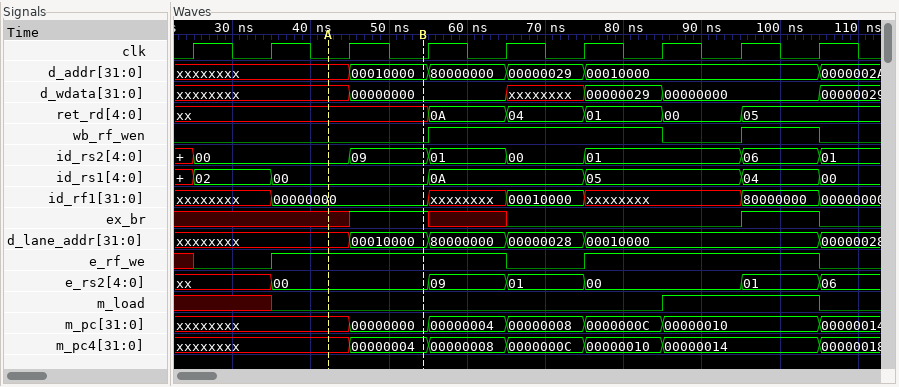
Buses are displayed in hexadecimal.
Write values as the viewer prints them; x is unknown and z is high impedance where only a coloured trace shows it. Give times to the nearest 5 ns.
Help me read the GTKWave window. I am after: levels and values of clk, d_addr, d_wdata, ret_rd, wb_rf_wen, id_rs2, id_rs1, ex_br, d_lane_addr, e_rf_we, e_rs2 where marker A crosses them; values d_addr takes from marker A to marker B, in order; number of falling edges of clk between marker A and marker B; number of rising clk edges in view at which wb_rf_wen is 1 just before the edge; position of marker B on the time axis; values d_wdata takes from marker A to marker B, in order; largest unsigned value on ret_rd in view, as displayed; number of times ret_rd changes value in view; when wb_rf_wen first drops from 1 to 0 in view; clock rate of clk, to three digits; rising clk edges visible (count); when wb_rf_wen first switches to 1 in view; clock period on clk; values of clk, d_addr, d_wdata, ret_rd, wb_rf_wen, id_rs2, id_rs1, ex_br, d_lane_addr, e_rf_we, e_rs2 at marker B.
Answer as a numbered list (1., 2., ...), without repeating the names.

1. clk=0, d_addr=xxxxxxxx, d_wdata=xxxxxxxx, ret_rd=xx, wb_rf_wen=0, id_rs2=00, id_rs1=00, ex_br=x, d_lane_addr=xxxxxxxx, e_rf_we=1, e_rs2=00
2. xxxxxxxx, 00010000
3. 1
4. 4
5. 55 ns
6. xxxxxxxx, 00000000
7. 0A
8. 5
9. 85 ns
10. 100 MHz
11. 9
12. 55 ns
13. 10 ns
14. clk=0, d_addr=00010000, d_wdata=00000000, ret_rd=xx, wb_rf_wen=0, id_rs2=09, id_rs1=00, ex_br=1, d_lane_addr=00010000, e_rf_we=1, e_rs2=00
